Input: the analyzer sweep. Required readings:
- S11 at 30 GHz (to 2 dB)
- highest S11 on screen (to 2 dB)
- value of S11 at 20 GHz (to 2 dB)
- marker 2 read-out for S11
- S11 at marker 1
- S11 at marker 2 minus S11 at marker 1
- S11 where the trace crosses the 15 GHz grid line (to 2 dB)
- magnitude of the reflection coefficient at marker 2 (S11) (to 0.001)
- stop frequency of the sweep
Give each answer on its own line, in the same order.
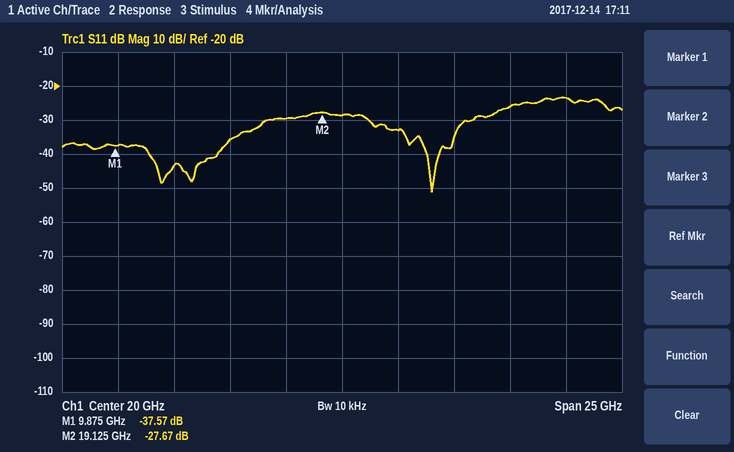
-24 dB
-24 dB
-28 dB
-27.67 dB
-37.57 dB
9.90 dB
-36 dB
0.041
32.5 GHz
